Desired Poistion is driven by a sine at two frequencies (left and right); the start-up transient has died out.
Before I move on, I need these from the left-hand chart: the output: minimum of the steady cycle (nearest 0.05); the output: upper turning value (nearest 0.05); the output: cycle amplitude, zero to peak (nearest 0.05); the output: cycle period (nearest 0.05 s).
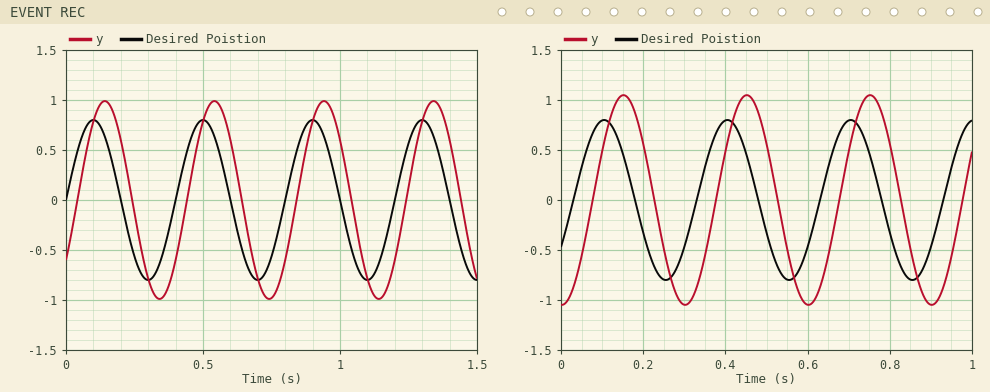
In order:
-1.00
1.00
1.00
0.40 s
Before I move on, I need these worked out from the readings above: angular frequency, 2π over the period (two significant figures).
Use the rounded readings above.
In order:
16 rad/s
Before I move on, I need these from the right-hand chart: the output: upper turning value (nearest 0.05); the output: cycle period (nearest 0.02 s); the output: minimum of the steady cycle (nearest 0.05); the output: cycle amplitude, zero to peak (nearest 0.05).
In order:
1.05
0.30 s
-1.05
1.05
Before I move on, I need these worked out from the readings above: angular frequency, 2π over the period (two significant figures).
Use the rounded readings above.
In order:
21 rad/s
